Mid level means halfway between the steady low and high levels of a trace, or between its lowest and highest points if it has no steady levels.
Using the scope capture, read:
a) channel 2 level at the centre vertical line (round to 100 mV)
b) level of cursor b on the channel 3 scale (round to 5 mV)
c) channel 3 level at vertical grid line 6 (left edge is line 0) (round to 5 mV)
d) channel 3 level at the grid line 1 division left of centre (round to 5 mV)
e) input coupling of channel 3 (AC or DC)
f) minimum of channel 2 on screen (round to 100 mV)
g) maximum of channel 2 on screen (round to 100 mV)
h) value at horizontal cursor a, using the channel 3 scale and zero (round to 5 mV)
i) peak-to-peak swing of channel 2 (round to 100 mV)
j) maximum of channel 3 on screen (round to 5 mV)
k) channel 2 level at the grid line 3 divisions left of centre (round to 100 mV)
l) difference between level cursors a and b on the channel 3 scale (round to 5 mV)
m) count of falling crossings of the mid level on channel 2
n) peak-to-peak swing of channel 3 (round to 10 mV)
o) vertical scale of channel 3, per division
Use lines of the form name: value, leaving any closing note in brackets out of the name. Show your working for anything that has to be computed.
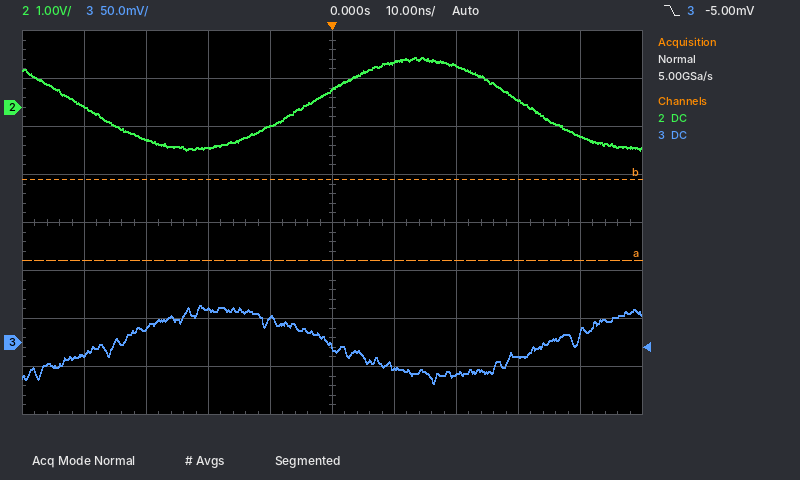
channel 2 level at the centre vertical line: 400 mV
level of cursor b on the channel 3 scale: 170 mV
channel 3 level at vertical grid line 6 (left edge is line 0): -25 mV
channel 3 level at the grid line 1 division left of centre: 25 mV
input coupling of channel 3: DC
minimum of channel 2 on screen: -900 mV
maximum of channel 2 on screen: 1.0 V
value at horizontal cursor a, using the channel 3 scale and zero: 85 mV
peak-to-peak swing of channel 2: 1.0 V − (-900 mV) = 1.9 V
maximum of channel 3 on screen: 40 mV
channel 2 level at the grid line 3 divisions left of centre: -700 mV
difference between level cursors a and b on the channel 3 scale: 85 mV
count of falling crossings of the mid level on channel 2: 2
peak-to-peak swing of channel 3: 80 mV
vertical scale of channel 3, per division: 50 mV
